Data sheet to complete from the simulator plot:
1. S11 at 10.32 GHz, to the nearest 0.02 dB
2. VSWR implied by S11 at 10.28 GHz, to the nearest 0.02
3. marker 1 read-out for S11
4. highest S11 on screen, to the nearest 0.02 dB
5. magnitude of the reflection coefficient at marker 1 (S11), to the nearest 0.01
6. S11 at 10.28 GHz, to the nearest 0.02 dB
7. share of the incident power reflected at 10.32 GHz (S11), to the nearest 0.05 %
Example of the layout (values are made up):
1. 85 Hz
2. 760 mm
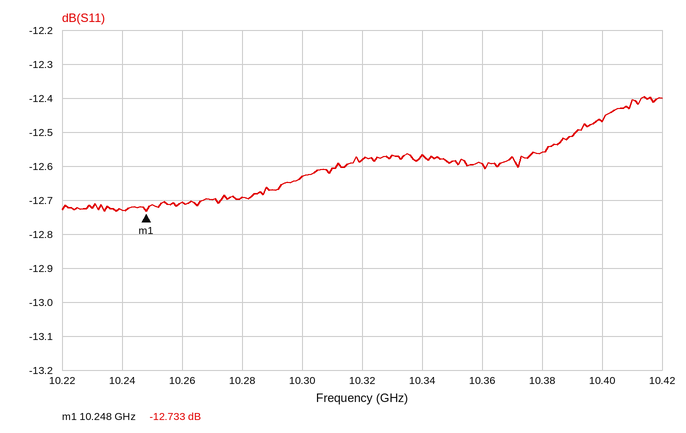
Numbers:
1. -12.58 dB
2. 1.60
3. -12.733 dB
4. -12.40 dB
5. 0.23
6. -12.70 dB
7. 5.50 %
